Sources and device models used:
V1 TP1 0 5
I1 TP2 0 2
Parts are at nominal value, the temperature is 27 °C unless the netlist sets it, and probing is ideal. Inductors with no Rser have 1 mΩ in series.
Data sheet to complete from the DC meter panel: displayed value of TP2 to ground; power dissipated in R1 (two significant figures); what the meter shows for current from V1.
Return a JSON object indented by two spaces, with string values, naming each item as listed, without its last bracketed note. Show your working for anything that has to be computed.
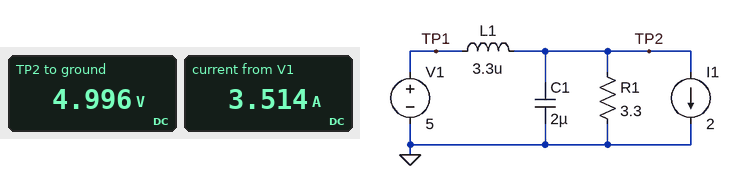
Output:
{
  "displayed value of TP2 to ground": "4.996 V",
  "power dissipated in R1": "(4.996 V)^2 / 3.3 Ω = 7.6 W",
  "what the meter shows for current from V1": "3.514 A"
}
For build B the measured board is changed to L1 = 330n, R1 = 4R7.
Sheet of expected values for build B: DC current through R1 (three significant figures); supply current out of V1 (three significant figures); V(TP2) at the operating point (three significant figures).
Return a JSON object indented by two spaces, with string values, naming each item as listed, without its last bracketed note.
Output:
{
  "DC current through R1": "1.06 A",
  "supply current out of V1": "3.06 A",
  "V(TP2) at the operating point": "5.00 V"
}
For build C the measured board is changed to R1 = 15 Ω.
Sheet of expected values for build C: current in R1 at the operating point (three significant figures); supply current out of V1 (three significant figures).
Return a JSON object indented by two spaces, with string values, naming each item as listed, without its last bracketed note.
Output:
{
  "current in R1 at the operating point": "333 mA",
  "supply current out of V1": "2.33 A"
}
